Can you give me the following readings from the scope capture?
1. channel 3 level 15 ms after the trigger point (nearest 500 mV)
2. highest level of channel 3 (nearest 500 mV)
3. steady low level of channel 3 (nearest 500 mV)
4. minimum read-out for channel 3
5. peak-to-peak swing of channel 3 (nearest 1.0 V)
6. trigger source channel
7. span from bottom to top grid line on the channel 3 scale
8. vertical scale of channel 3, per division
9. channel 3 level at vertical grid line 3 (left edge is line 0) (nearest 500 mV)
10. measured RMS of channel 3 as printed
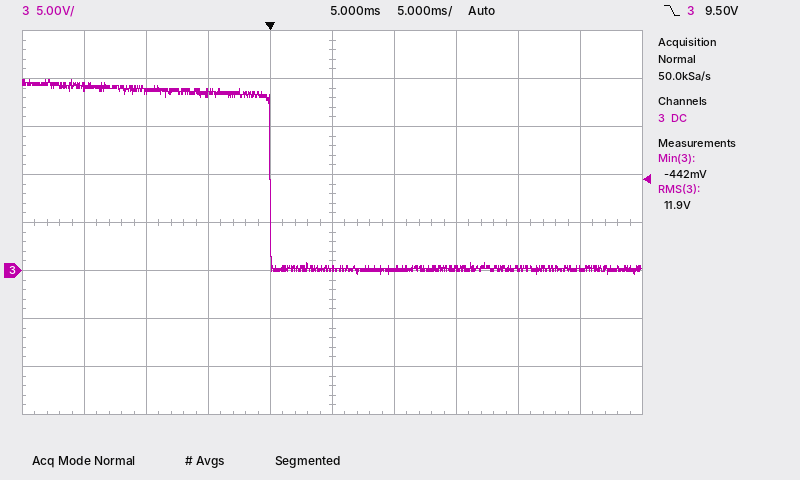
0.0 V
20.0 V
0.0 V
-442 mV
20.0 V
channel 3
40 V
5 V
18.5 V
11.9 V
